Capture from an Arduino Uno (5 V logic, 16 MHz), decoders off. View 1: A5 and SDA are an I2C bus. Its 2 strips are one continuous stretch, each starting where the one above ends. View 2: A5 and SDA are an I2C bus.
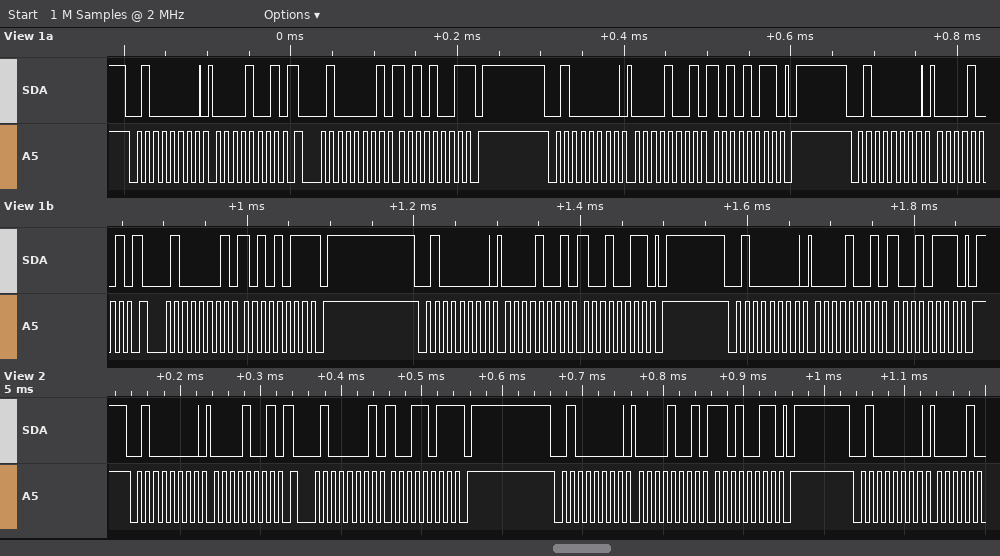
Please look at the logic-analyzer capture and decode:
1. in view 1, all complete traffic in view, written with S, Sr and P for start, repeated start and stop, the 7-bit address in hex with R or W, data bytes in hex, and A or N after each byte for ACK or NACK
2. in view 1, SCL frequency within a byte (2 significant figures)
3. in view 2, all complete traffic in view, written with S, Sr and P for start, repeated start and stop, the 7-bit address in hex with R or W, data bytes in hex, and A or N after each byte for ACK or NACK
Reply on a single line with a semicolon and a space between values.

S 20W A 09 A Sr 20R A A9 N P S 20W A 09 A AB A P S 20W A 09 A Sr 20R A AB N P S 20W A 09 A 93 A P S 20W A 09 A 97 A P; 100 kHz; S 20W A 09 A Sr 20R A 9B N P S 20W A 09 A D3 A P S 20W A
